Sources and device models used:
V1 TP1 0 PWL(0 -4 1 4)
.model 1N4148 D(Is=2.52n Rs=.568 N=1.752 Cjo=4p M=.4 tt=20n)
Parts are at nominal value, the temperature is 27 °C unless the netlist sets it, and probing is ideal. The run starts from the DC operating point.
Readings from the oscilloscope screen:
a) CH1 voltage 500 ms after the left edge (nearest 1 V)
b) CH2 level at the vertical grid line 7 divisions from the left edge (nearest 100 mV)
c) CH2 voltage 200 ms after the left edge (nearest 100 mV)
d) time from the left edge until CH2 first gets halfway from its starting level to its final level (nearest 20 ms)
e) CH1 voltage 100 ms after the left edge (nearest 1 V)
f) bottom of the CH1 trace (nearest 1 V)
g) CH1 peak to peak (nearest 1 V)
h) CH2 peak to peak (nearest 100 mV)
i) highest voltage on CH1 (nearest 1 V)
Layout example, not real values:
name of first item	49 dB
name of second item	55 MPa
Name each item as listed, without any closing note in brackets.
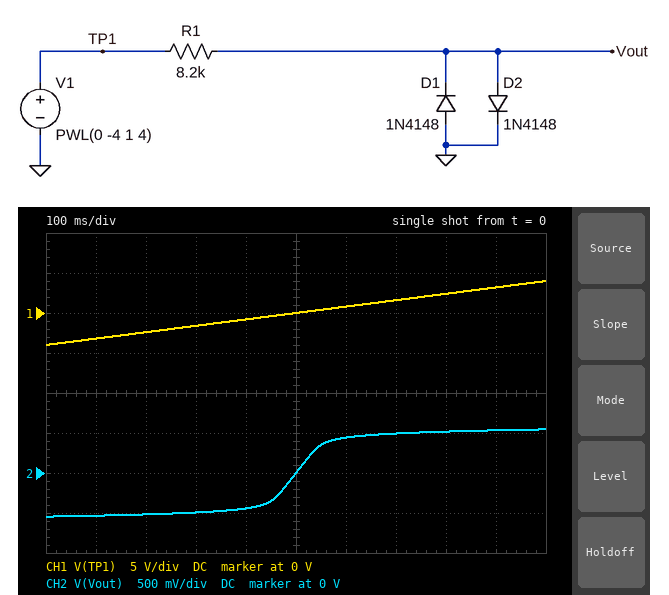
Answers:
CH1 voltage 500 ms after the left edge	0 V
CH2 level at the vertical grid line 7 divisions from the left edge	500 mV
CH2 voltage 200 ms after the left edge	-500 mV
time from the left edge until CH2 first gets halfway from its starting level to its final level	500 ms
CH1 voltage 100 ms after the left edge	-3 V
bottom of the CH1 trace	-4 V
CH1 peak to peak	8 V
CH2 peak to peak	1.1 V
highest voltage on CH1	4 V
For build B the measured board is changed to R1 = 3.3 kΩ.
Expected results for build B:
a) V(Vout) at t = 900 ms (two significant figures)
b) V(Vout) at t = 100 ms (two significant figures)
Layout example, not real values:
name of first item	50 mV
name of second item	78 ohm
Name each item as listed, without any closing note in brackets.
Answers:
V(Vout) at t = 900 ms	570 mV
V(Vout) at t = 100 ms	-570 mV
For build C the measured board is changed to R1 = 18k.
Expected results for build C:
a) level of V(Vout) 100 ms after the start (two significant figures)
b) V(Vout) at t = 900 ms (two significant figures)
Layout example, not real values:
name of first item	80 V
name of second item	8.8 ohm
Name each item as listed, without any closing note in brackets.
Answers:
level of V(Vout) 100 ms after the start	-500 mV
V(Vout) at t = 900 ms	500 mV
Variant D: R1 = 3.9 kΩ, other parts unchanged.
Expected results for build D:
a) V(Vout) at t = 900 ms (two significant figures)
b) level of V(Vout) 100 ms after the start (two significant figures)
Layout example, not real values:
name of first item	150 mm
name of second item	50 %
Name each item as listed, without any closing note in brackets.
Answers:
V(Vout) at t = 900 ms	570 mV
level of V(Vout) 100 ms after the start	-570 mV
